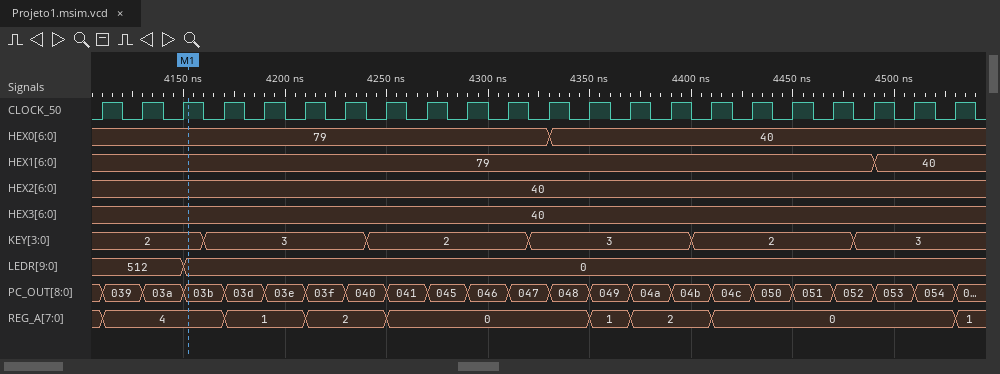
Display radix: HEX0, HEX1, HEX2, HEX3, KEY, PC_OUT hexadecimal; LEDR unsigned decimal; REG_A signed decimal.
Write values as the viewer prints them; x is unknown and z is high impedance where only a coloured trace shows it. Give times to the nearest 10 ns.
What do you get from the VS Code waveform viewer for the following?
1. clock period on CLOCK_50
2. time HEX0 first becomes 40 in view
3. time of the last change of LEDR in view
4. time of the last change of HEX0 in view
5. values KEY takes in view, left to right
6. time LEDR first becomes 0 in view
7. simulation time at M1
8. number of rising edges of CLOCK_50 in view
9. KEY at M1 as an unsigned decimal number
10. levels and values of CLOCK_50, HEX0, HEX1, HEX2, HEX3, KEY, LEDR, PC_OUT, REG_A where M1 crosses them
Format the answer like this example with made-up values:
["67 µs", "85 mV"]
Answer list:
["20 ns", "4330 ns", "4150 ns", "4330 ns", "2, 3, 2, 3, 2, 3", "4150 ns", "4150 ns", "22", "2", "CLOCK_50=1, HEX0=79, HEX1=79, HEX2=40, HEX3=40, KEY=2, LEDR=0, PC_OUT=03b, REG_A=4"]
